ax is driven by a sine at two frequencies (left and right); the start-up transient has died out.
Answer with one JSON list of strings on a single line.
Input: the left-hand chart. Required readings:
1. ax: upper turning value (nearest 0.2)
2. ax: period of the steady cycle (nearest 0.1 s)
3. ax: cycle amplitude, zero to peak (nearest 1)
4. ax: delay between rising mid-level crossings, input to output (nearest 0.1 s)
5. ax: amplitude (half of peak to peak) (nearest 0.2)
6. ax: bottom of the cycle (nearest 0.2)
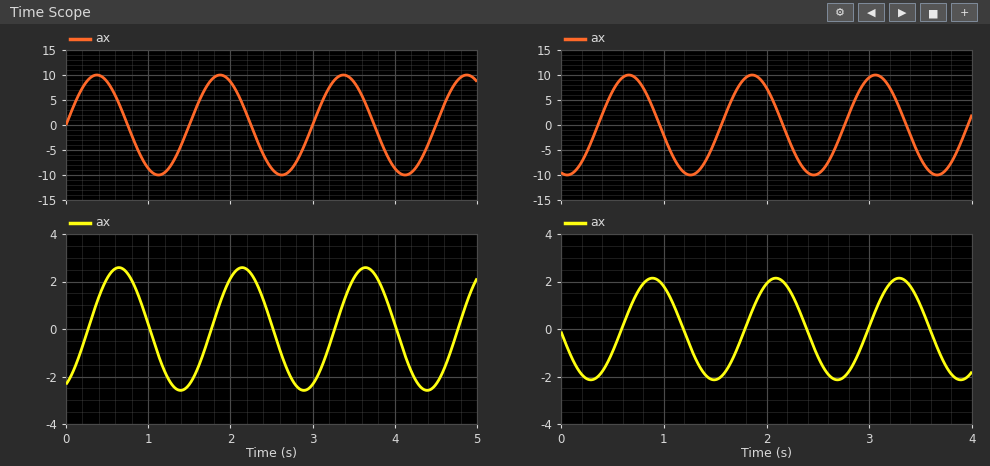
["2.6", "1.5 s", "10", "0.3 s", "2.6", "-2.6"]
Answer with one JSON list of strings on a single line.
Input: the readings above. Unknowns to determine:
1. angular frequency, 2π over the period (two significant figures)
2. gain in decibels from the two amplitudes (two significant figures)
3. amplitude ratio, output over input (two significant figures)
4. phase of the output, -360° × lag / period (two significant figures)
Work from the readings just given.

["4.2 rad/s", "-12 dB", "0.26", "-72°"]
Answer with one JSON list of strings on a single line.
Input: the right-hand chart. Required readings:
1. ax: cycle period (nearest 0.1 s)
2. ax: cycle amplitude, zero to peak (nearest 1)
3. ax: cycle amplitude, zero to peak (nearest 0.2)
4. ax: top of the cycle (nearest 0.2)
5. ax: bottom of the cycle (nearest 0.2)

["1.2 s", "10", "2.2", "2.2", "-2.2"]
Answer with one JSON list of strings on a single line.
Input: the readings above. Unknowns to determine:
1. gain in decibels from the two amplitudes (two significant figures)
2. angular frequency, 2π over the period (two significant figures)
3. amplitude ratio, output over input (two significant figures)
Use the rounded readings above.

["-13 dB", "5.2 rad/s", "0.22"]
